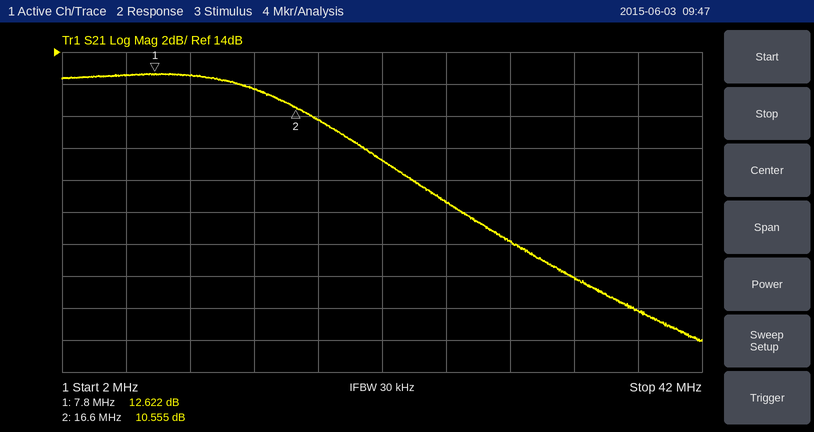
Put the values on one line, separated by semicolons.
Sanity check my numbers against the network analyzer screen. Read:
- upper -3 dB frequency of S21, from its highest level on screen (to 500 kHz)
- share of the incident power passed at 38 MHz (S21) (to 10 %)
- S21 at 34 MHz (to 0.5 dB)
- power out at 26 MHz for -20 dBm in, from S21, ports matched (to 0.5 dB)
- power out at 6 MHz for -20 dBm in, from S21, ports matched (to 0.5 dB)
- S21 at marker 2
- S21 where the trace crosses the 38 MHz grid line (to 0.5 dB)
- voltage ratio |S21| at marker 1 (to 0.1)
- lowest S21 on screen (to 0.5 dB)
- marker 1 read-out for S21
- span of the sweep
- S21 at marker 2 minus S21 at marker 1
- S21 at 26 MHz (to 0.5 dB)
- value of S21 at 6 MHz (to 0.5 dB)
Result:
18.0 MHz; 60 %; 0.0 dB; -15.5 dBm; -7.5 dBm; 10.555 dB; -2.0 dB; 4.3; -4.0 dB; 12.622 dB; 40 MHz; -2.067 dB; 4.5 dB; 12.5 dB
